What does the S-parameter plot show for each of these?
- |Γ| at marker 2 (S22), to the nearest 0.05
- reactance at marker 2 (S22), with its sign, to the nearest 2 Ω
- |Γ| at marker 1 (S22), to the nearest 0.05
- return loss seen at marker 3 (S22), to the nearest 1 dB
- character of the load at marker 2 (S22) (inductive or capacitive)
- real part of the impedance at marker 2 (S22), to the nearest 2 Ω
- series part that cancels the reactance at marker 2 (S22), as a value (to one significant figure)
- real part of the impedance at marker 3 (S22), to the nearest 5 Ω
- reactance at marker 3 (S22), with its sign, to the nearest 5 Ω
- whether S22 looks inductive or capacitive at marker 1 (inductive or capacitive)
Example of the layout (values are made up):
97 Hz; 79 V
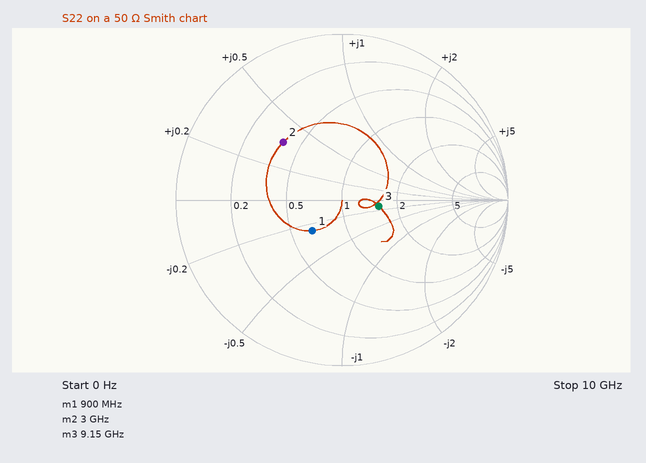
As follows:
0.50; +18 Ω; 0.25; 13 dB; inductive; 20 Ω; 3 pF; 80 Ω; -5 Ω; capacitive
